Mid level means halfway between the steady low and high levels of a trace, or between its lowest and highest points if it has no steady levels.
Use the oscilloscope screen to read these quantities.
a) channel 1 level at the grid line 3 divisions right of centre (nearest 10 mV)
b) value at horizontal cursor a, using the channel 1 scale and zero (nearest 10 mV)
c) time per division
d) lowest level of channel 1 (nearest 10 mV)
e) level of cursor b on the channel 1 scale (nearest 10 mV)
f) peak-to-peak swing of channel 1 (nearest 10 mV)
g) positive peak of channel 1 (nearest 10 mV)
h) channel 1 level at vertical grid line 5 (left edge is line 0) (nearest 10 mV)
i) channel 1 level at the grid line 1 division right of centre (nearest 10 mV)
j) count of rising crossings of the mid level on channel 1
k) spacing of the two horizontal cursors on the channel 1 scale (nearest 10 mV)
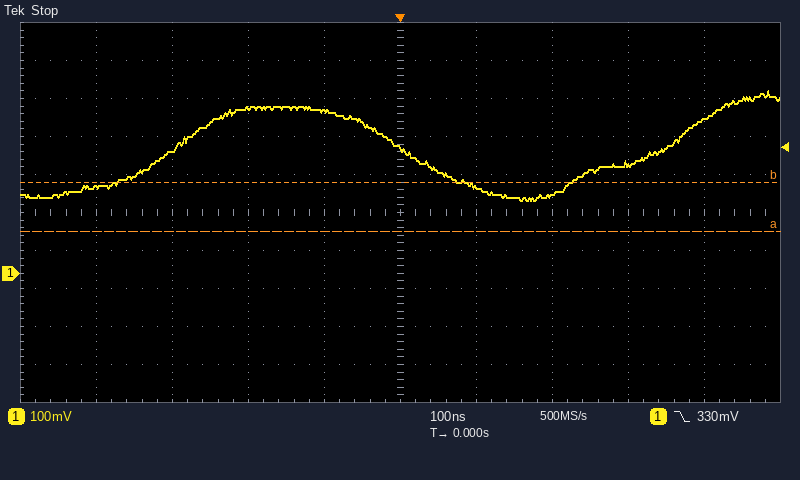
290 mV
110 mV
100 ns
190 mV
240 mV
290 mV
480 mV
330 mV
230 mV
2
130 mV
